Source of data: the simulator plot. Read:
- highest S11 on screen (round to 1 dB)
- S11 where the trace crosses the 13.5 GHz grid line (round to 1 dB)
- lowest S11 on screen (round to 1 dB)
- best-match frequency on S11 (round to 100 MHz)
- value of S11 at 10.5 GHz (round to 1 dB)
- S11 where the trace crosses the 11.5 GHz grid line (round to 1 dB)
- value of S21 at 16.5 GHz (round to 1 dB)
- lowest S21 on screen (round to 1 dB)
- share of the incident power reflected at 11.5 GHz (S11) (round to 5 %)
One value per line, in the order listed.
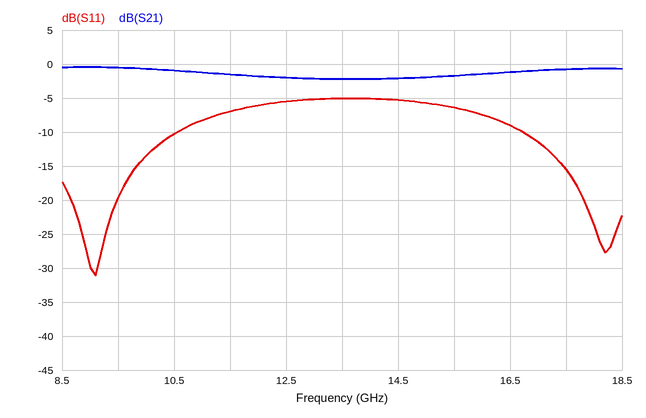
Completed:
-5 dB
-5 dB
-31 dB
9.1 GHz
-10 dB
-7 dB
-1 dB
-2 dB
20 %
